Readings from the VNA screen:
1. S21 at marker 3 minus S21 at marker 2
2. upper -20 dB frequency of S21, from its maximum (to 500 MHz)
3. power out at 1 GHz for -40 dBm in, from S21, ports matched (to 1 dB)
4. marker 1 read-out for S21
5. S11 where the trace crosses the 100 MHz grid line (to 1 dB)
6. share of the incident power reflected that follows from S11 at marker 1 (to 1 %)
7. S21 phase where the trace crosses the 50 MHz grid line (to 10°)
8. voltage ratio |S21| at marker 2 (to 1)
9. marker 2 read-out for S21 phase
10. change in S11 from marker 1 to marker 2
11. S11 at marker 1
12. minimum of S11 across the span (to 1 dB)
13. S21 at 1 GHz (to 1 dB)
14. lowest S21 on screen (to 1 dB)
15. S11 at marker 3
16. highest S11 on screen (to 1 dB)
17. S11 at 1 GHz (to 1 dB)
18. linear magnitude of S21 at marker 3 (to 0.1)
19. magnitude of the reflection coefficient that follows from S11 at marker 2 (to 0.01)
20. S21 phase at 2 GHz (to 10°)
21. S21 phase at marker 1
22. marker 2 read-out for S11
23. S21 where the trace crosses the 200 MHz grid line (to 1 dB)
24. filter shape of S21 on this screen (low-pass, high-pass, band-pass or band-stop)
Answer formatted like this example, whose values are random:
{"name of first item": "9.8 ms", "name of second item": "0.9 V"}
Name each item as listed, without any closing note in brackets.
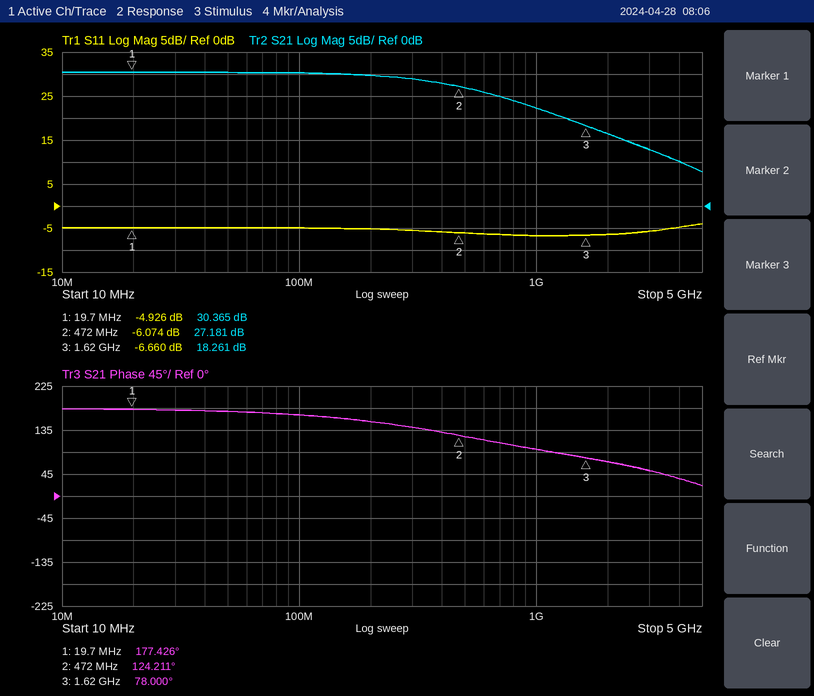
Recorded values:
{"S21 at marker 3 minus S21 at marker 2": "-8.920 dB", "upper -20 dB frequency of S21, from its maximum": "4.0 GHz", "power out at 1 GHz for -40 dBm in, from S21, ports matched": "-18 dBm", "marker 1 read-out for S21": "30.365 dB", "S11 where the trace crosses the 100 MHz grid line": "-5 dB", "share of the incident power reflected that follows from S11 at marker 1": "32 %", "S21 phase where the trace crosses the 50 MHz grid line": "170°", "voltage ratio |S21| at marker 2": "23", "marker 2 read-out for S21 phase": "124.211°", "change in S11 from marker 1 to marker 2": "-1.148 dB", "S11 at marker 1": "-4.926 dB", "minimum of S11 across the span": "-7 dB", "S21 at 1 GHz": "22 dB", "lowest S21 on screen": "8 dB", "S11 at marker 3": "-6.660 dB", "highest S11 on screen": "-4 dB", "S11 at 1 GHz": "-7 dB", "linear magnitude of S21 at marker 3": "8.2", "magnitude of the reflection coefficient that follows from S11 at marker 2": "0.50", "S21 phase at 2 GHz": "70°", "S21 phase at marker 1": "177.426°", "marker 2 read-out for S11": "-6.074 dB", "S21 where the trace crosses the 200 MHz grid line": "30 dB", "filter shape of S21 on this screen": "low-pass"}
